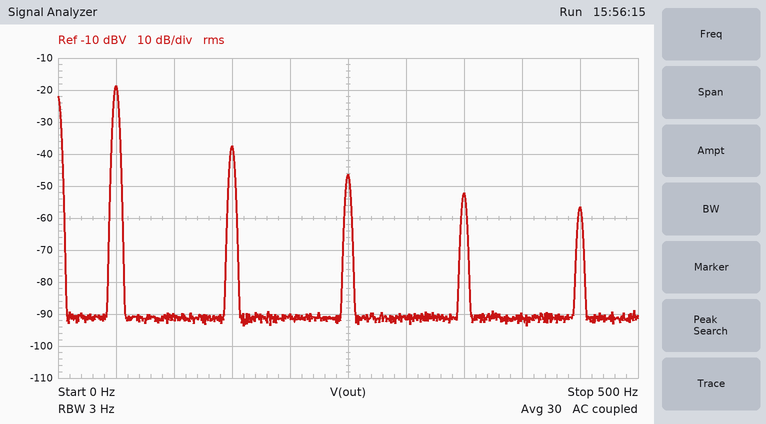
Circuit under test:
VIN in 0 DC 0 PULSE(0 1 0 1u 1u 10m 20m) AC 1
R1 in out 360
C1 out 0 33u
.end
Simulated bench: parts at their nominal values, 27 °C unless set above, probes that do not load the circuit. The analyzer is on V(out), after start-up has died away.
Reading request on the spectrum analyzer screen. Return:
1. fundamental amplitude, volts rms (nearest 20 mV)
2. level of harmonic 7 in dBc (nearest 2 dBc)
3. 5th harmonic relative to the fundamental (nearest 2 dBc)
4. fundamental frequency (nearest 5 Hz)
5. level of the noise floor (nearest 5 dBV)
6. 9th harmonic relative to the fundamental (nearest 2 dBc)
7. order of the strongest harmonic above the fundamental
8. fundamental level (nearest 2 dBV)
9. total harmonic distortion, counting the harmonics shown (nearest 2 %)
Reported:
120 mV
-34 dBc
-28 dBc
50 Hz
-90 dBV
-38 dBc
3
-18 dBV
12 %
